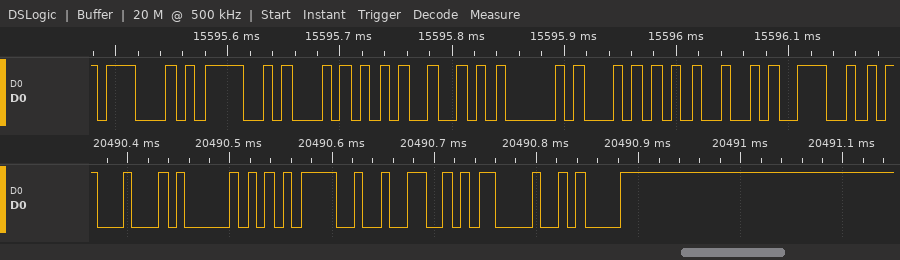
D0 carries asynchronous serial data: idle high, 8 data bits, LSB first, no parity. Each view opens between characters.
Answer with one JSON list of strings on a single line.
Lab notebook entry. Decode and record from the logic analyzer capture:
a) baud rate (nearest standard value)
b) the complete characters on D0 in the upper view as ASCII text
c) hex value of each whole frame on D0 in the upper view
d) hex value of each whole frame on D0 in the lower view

["115200 baud", "\"GOTIATIN\"", "47, 4F, 54, 49, 41, 54, 49, 4E", "44, 50, 3D, 32, 0D, 0A"]
